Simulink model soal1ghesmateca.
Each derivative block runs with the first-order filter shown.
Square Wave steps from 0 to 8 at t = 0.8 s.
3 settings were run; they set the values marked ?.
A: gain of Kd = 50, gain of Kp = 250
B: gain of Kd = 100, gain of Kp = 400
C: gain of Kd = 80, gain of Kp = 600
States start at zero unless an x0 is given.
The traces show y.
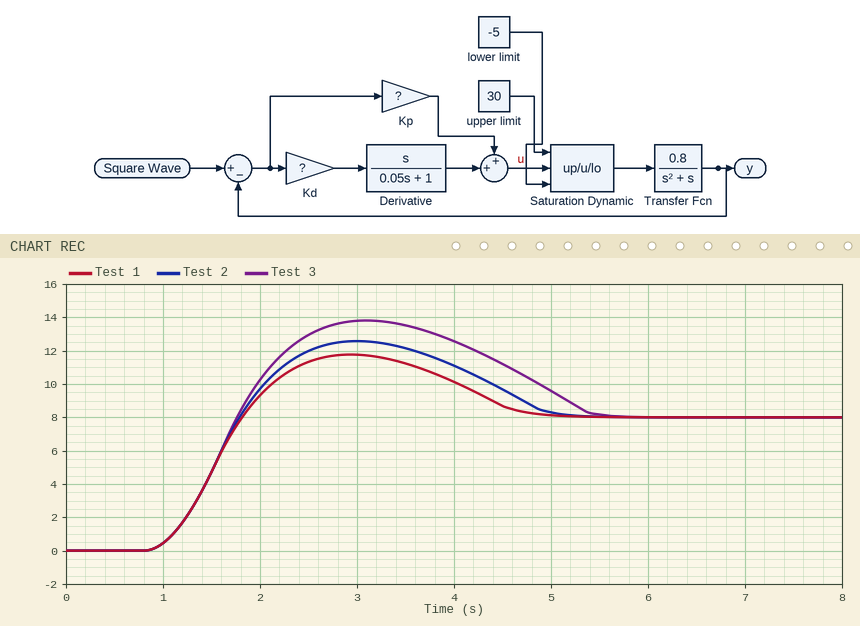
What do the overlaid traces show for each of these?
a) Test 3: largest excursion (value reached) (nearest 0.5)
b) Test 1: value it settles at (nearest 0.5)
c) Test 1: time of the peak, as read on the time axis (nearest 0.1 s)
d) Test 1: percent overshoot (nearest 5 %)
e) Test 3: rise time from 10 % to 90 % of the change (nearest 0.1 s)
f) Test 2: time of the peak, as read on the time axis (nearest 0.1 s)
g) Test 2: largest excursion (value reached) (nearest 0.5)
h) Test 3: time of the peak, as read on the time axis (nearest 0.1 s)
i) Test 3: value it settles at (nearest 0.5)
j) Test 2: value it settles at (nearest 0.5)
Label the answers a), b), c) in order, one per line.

a) 14.0
b) 8.0
c) 2.9 s
d) 45 %
e) 0.6 s
f) 3.0 s
g) 12.5
h) 3.1 s
i) 8.0
j) 8.0
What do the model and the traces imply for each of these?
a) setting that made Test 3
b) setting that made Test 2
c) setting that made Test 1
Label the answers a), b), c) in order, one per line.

a) C
b) A
c) B
